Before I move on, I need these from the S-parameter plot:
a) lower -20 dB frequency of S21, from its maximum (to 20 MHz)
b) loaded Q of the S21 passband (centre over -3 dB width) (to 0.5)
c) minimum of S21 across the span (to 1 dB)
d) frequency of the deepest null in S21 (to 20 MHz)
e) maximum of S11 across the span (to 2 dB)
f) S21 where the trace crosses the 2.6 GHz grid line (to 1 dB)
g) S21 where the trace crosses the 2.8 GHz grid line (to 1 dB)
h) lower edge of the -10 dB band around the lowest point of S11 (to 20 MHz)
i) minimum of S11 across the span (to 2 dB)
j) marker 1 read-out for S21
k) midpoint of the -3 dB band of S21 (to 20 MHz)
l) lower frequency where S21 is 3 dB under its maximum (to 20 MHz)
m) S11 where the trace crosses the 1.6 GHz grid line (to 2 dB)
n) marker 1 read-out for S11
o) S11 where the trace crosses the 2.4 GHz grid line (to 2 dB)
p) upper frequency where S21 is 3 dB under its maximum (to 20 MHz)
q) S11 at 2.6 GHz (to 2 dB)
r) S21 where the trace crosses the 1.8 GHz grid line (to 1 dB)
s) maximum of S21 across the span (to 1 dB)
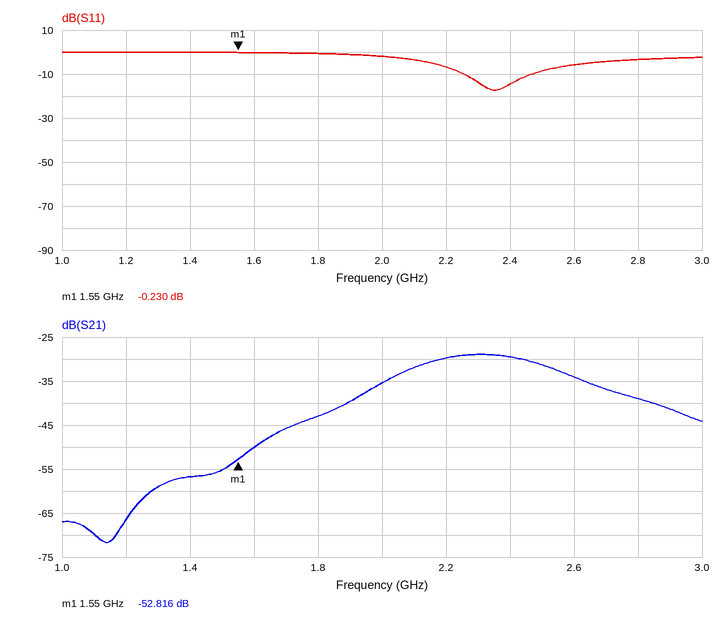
1.62 GHz
5.5
-72 dB
1.14 GHz
0 dB
-34 dB
-39 dB
2.26 GHz
-18 dB
-52.816 dB
2.32 GHz
2.10 GHz
0 dB
-0.230 dB
-14 dB
2.52 GHz
-6 dB
-43 dB
-29 dB
